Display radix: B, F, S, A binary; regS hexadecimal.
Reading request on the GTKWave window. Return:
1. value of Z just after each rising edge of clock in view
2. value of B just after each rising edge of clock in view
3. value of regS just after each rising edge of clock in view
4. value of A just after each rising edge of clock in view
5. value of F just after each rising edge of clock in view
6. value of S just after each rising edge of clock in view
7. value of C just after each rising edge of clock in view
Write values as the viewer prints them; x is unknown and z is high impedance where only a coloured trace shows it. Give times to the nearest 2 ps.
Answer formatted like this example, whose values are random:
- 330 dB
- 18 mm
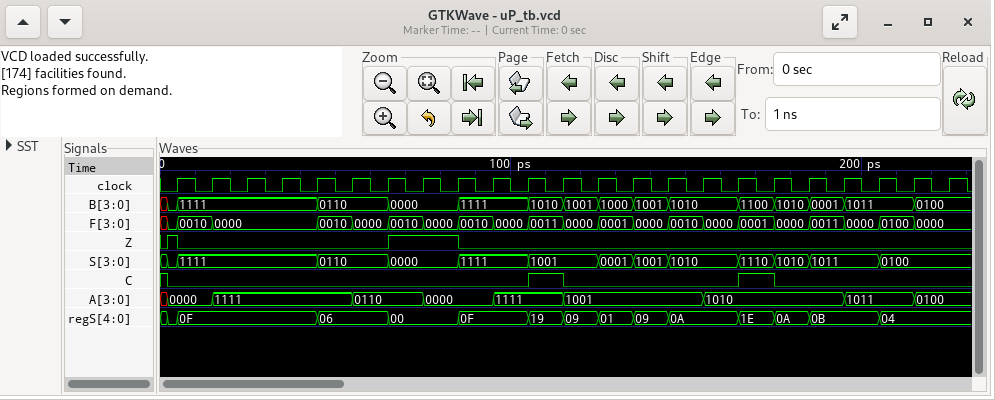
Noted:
- 0 0 0 0 0 0 1 1 0 0 0 0 0 0 0 0 0 0 0 0 0 0 0
- 1111, 1111, 1111, 1111, 0110, 0110, 0000, 0000, 1111, 1111, 1010, 1001, 1000, 1001, 1010, 1010, 1100, 1010, 0001, 1011, 1011, 0100, 0100
- 0F, 0F, 0F, 0F, 06, 06, 00, 00, 0F, 0F, 19, 09, 01, 09, 0A, 0A, 1E, 0A, 0B, 0B, 04, 04, 04
- 0000, 1111, 1111, 1111, 1111, 0110, 0110, 0000, 0000, 1111, 1111, 1001, 1001, 1001, 1001, 1010, 1010, 1010, 1010, 1011, 1011, 0100, 0100
- 0010, 0000, 0000, 0000, 0010, 0000, 0010, 0000, 0010, 0000, 0011, 0000, 0001, 0000, 0010, 0000, 0001, 0000, 0011, 0000, 0100, 0000, 0000
- 1111, 1111, 1111, 1111, 0110, 0110, 0000, 0000, 1111, 1111, 1001, 1001, 0001, 1001, 1010, 1010, 1110, 1010, 1011, 1011, 0100, 0100, 0100
- 0 0 0 0 0 0 0 0 0 0 1 0 0 0 0 0 1 0 0 0 0 0 0
